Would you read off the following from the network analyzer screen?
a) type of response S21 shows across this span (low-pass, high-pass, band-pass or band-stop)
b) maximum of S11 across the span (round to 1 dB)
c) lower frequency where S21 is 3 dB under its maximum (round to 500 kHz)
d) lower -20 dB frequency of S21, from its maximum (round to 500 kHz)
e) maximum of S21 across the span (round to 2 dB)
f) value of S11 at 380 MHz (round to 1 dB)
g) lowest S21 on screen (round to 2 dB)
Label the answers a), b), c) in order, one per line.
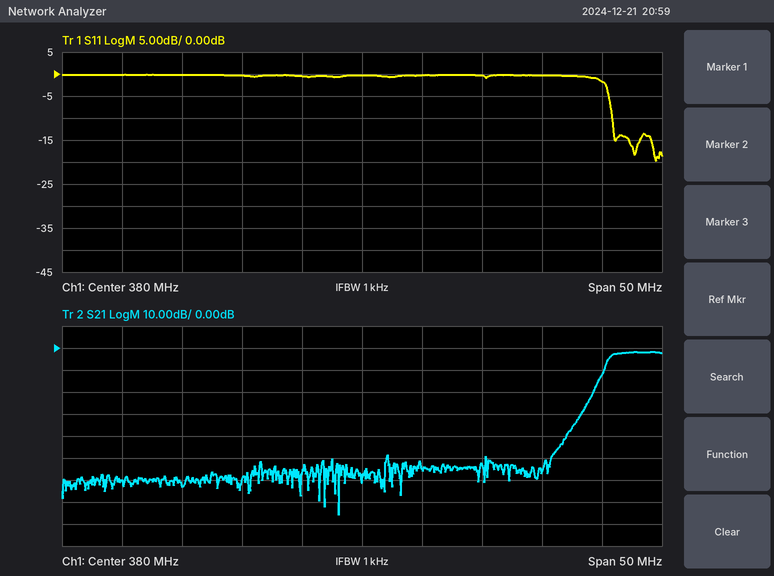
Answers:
a) high-pass
b) 0 dB
c) 400.5 MHz
d) 399.0 MHz
e) -2 dB
f) 0 dB
g) -76 dB
